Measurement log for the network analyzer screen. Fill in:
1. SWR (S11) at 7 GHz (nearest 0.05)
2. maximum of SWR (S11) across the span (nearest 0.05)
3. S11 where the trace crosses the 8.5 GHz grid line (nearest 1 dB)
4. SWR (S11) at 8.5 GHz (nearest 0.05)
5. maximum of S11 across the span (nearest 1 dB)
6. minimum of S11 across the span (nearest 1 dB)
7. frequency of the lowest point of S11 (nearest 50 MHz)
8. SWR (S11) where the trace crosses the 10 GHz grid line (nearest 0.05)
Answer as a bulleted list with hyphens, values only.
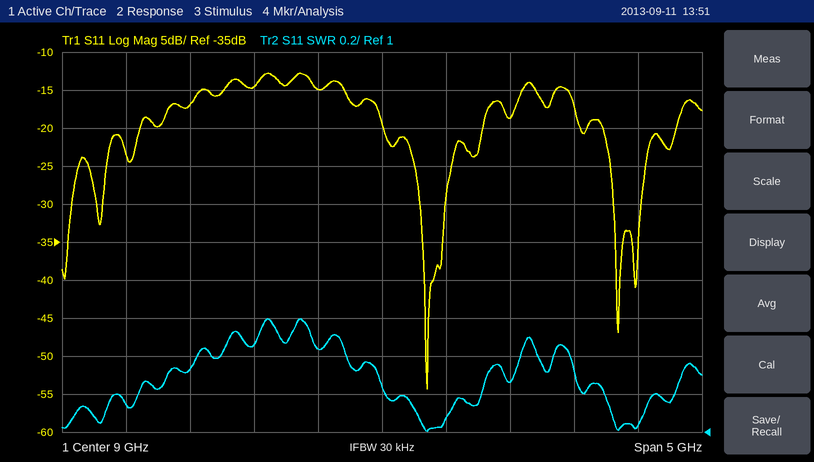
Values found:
- 1.15
- 1.60
- -15 dB
- 1.45
- -13 dB
- -54 dB
- 9.35 GHz
- 1.25
